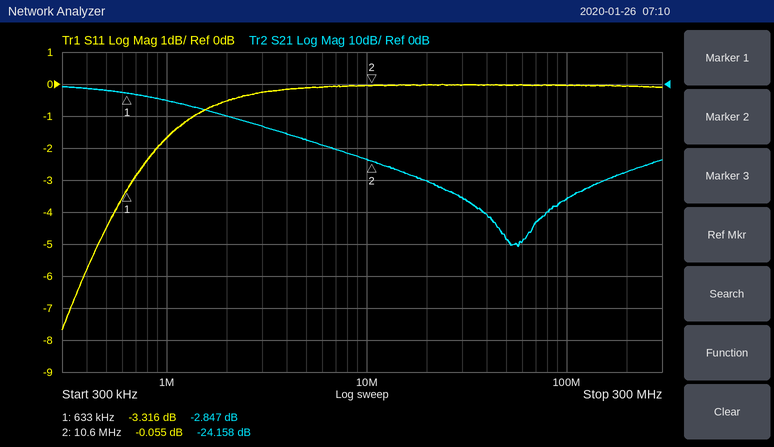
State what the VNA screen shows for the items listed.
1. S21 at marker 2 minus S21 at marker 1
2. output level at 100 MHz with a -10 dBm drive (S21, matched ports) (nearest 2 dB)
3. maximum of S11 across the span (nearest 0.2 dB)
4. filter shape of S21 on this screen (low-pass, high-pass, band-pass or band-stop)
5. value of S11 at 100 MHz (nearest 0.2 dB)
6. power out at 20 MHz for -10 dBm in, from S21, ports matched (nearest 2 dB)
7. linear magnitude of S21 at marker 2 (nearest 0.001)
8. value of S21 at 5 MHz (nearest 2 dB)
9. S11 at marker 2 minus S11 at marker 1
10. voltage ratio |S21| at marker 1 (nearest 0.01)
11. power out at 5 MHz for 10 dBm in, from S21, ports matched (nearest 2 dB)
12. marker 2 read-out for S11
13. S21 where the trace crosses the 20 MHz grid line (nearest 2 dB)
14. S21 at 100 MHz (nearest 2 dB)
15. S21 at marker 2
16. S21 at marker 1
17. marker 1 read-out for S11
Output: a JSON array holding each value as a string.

["-21.311 dB", "-46 dBm", "0.0 dB", "low-pass", "0.0 dB", "-40 dBm", "0.062", "-18 dB", "3.261 dB", "0.72", "-8 dBm", "-0.055 dB", "-30 dB", "-36 dB", "-24.158 dB", "-2.847 dB", "-3.316 dB"]
